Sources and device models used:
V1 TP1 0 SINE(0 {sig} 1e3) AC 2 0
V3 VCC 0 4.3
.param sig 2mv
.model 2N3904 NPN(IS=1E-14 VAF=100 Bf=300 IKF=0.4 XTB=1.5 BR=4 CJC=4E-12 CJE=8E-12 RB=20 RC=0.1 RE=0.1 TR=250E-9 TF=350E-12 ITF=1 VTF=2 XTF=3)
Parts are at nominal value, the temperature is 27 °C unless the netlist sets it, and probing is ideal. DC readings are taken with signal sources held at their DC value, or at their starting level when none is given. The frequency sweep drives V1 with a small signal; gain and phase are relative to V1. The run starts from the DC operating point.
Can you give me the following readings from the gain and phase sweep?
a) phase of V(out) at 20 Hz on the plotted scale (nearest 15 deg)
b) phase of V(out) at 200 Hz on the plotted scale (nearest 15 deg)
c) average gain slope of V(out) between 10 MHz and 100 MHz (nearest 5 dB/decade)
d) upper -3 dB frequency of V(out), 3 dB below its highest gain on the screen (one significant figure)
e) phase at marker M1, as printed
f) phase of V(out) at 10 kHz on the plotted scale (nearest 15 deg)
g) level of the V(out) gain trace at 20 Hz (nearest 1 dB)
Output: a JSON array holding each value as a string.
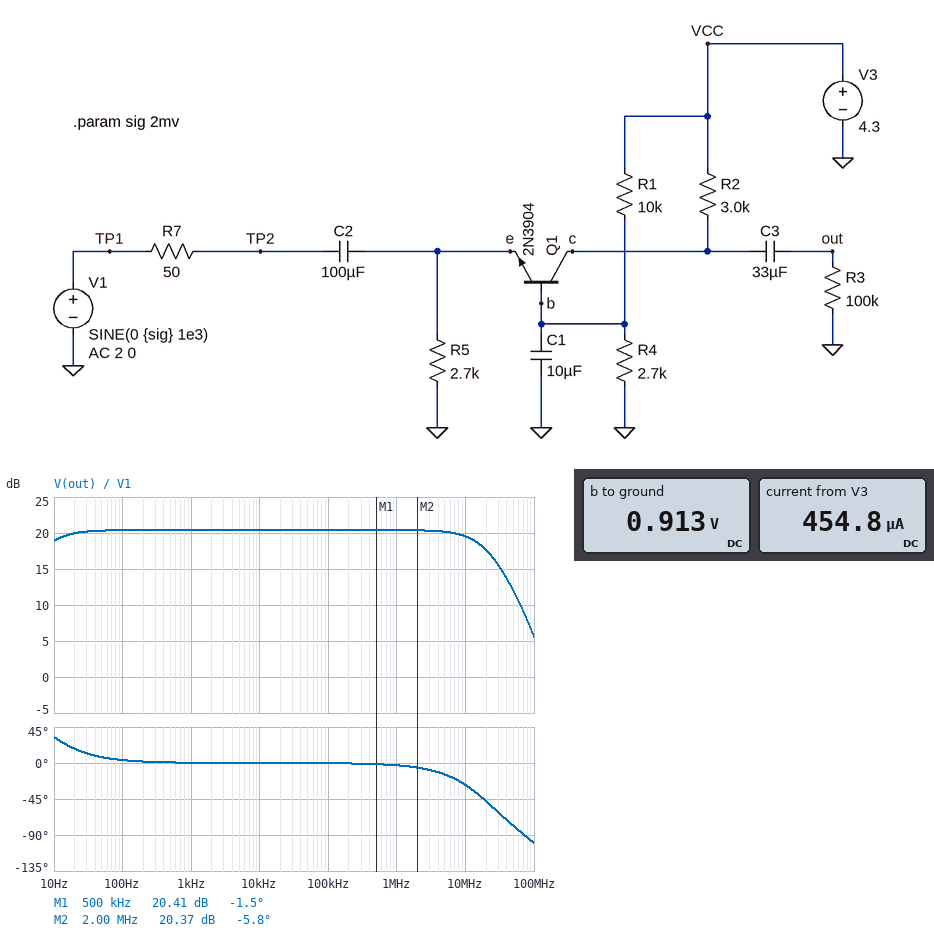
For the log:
["15 deg", "0 deg", "-15 dB/decade", "20 MHz", "-1.5 deg", "0 deg", "20 dB"]
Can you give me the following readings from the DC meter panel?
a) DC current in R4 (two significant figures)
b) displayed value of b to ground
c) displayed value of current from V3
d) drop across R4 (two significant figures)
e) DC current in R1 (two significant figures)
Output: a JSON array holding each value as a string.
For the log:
["340 µA", "0.913 V", "454.8 µA", "910 mV", "340 µA"]
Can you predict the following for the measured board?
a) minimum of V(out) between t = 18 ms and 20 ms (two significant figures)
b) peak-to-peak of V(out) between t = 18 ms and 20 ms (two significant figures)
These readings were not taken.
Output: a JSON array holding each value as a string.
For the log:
["-21 mV", "42 mV"]
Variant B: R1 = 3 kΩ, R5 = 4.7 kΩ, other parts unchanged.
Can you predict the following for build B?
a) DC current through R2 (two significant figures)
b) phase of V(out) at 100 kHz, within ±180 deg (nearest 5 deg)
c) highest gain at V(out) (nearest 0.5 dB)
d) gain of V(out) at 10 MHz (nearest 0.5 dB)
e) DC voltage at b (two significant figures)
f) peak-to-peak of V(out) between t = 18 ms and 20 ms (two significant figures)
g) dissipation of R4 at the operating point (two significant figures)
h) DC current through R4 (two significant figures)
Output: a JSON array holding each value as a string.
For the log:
["300 µA", "0 deg", "26.5 dB", "25.0 dB", "2.0 V", "84 mV", "1.5 mW", "750 µA"]
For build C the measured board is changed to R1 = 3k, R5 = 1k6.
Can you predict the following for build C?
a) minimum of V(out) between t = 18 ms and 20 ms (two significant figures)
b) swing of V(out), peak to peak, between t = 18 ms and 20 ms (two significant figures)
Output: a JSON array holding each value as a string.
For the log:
["-71 mV", "140 mV"]
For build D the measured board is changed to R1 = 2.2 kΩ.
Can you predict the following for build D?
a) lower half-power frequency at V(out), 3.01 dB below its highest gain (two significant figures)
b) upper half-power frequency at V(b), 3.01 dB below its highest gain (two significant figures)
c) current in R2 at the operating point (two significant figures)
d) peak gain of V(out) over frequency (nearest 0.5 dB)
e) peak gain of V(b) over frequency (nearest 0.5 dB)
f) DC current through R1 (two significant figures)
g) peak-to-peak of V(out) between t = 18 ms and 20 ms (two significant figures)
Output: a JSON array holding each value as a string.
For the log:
["18 Hz", "37 Hz", "640 µA", "30.0 dB", "-34.5 dB", "880 µA", "130 mV"]
